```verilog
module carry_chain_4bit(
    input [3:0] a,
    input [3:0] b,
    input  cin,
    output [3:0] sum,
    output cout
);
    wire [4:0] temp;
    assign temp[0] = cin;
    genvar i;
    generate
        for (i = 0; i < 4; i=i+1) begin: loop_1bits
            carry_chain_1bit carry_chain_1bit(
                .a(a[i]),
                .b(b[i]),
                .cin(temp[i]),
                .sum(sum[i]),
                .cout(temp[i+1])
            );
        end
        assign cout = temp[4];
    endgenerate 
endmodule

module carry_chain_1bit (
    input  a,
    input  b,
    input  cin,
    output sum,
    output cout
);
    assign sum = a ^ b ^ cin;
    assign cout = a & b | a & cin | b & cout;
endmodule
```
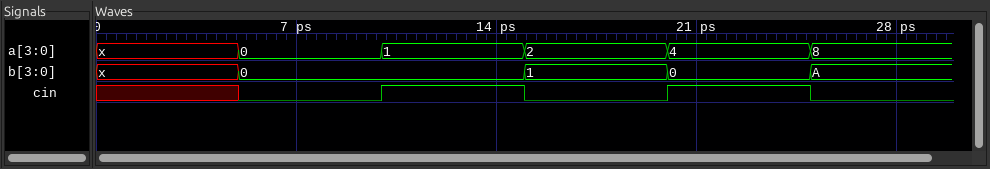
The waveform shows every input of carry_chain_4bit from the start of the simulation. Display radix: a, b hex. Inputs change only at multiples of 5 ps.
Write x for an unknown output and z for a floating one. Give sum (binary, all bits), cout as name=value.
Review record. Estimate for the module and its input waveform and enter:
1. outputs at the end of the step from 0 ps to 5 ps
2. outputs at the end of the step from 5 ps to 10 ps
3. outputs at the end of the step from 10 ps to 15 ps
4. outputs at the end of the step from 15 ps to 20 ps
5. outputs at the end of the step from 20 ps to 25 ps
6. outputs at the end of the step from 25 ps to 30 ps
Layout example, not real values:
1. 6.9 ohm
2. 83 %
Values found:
1. sum=x, cout=x
2. sum=0000, cout=0
3. sum=0010, cout=0
4. sum=0101, cout=0
5. sum=0101, cout=0
6. sum=0010, cout=1
